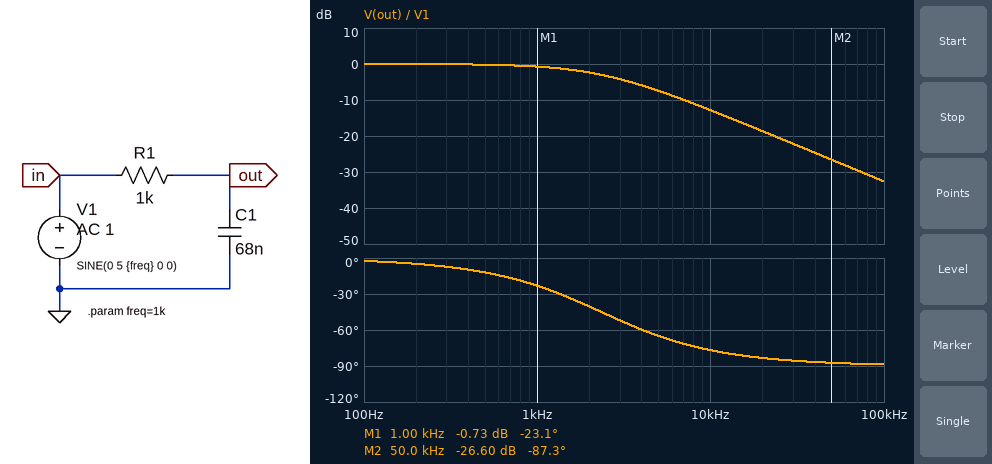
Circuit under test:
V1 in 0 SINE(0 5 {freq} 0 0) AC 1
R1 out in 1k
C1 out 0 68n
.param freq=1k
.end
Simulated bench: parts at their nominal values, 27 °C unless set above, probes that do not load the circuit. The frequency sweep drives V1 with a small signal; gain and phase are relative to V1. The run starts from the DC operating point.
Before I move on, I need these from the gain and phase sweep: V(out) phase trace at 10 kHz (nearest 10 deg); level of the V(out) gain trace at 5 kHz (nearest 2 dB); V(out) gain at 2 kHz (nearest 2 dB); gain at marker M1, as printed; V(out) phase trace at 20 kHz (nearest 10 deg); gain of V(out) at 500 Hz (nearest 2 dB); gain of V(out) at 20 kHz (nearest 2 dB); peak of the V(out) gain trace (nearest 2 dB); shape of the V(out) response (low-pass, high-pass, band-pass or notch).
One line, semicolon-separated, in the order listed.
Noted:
-80 deg; -8 dB; -2 dB; -0.73 dB; -80 deg; 0 dB; -18 dB; 0 dB; low-pass
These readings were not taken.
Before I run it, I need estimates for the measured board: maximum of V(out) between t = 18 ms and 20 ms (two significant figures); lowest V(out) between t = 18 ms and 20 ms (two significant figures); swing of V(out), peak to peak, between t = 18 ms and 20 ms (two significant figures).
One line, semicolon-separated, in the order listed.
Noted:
4.6 V; -4.6 V; 9.2 V
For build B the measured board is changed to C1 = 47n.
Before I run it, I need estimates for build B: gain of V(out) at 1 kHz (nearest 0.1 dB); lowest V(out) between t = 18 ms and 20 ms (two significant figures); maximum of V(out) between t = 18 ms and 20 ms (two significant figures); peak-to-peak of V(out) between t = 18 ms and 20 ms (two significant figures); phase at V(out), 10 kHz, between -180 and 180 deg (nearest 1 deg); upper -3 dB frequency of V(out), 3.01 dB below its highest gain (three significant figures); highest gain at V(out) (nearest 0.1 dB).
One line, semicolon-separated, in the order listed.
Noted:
-0.4 dB; -4.8 V; 4.8 V; 9.6 V; -71 deg; 3.39 kHz; 0 dB
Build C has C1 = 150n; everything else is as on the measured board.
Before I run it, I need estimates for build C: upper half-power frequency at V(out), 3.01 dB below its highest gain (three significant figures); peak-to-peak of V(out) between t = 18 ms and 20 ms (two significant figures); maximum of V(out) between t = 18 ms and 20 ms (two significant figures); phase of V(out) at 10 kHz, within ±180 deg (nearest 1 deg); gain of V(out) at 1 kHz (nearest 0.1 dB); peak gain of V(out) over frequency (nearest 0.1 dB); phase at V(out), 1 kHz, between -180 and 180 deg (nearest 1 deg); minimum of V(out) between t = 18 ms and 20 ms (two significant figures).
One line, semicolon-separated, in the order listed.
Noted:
1.06 kHz; 7.3 V; 3.6 V; -84 deg; -2.8 dB; 0 dB; -43 deg; -3.6 V
